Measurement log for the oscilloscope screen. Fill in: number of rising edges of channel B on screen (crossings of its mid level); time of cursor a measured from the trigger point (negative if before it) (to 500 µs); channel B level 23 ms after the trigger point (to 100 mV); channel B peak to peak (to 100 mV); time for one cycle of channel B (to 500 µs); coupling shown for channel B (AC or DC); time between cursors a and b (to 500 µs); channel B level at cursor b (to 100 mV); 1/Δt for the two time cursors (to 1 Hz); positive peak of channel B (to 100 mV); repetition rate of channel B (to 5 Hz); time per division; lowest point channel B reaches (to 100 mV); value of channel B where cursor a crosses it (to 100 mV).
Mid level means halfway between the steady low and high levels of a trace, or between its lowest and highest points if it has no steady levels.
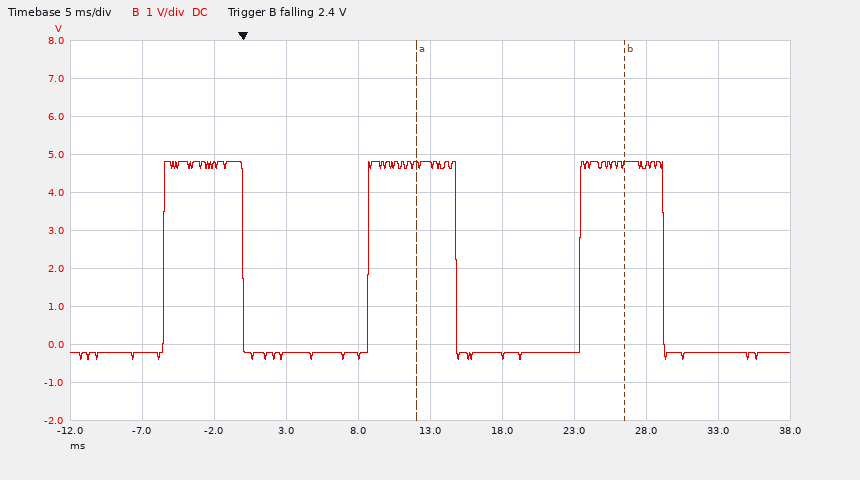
3
+12.0 ms
-200 mV
5.2 V
14.5 ms
DC
14.5 ms
4.7 V
69 Hz
4.8 V
70 Hz
5 ms
-400 mV
4.7 V
